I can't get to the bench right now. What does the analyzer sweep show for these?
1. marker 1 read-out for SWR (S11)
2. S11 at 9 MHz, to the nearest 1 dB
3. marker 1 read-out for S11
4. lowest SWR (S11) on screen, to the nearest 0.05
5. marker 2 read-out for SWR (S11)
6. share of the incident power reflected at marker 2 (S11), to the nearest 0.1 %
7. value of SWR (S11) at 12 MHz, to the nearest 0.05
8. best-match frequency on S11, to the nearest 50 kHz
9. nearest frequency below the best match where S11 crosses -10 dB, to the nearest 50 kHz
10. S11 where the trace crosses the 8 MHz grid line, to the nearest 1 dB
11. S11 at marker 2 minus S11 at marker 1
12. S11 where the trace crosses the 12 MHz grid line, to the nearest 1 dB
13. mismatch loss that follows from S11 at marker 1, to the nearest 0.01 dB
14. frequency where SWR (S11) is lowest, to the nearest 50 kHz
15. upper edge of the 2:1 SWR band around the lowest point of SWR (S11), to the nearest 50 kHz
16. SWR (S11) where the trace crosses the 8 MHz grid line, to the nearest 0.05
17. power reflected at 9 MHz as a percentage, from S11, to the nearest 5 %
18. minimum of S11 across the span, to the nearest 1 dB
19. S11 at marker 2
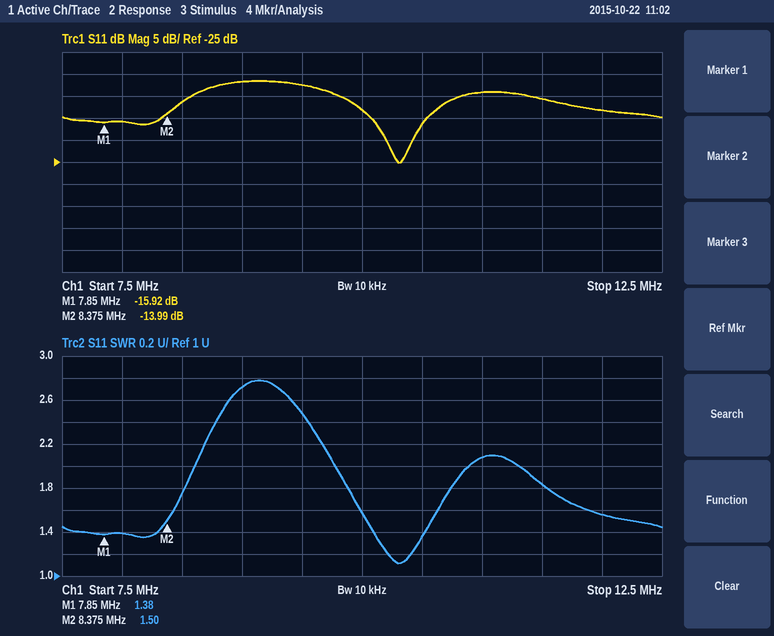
1.38
-7 dB
-15.92 dB
1.10
1.50
4.0 %
1.55
10.30 MHz
9.80 MHz
-16 dB
1.93 dB
-13 dB
0.11 dB
10.30 MHz
10.90 MHz
1.40
20 %
-25 dB
-13.99 dB
